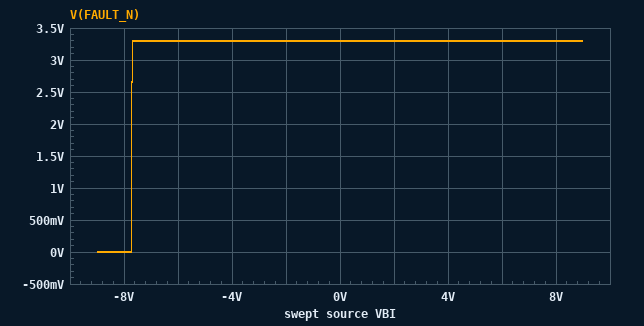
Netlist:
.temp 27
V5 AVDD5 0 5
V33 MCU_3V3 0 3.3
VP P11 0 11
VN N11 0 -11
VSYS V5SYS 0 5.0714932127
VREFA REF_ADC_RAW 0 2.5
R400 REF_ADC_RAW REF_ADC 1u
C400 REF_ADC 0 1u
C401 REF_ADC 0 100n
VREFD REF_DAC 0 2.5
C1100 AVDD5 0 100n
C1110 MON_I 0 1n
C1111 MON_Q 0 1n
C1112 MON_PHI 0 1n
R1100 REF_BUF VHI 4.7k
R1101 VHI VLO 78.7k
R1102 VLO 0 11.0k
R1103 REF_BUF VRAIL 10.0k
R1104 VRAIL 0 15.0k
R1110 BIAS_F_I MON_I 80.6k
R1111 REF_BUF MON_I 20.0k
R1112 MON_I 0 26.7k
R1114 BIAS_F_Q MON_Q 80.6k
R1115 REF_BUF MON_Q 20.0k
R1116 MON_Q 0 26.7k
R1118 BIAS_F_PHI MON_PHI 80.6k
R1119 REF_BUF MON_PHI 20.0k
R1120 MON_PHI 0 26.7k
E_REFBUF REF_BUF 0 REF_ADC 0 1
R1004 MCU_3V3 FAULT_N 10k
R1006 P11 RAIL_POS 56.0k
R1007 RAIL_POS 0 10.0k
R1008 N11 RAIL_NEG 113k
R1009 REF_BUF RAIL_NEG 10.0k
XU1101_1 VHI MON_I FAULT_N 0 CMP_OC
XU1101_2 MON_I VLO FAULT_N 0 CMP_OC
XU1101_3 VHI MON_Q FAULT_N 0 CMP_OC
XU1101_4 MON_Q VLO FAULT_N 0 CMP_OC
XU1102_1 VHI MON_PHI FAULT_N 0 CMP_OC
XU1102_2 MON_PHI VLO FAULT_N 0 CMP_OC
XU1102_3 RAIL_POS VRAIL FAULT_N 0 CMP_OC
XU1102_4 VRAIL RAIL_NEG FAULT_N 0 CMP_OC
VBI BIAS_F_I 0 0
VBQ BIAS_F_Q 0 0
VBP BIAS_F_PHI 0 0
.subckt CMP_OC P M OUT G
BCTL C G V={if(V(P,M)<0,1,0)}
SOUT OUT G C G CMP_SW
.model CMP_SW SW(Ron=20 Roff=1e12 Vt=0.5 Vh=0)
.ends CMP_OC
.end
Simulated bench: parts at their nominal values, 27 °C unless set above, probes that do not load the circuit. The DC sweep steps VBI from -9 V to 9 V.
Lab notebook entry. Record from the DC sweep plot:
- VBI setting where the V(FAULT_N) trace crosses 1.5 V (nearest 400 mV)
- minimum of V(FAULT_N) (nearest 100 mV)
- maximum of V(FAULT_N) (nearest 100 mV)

-7.6 V
0 V
3.3 V
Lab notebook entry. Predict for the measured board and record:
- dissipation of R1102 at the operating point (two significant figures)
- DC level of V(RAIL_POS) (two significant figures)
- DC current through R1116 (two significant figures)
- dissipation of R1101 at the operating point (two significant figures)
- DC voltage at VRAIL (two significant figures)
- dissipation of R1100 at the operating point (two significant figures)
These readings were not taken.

7.7 µW
1.7 V
47 µA
55 µW
1.5 V
3.3 µW
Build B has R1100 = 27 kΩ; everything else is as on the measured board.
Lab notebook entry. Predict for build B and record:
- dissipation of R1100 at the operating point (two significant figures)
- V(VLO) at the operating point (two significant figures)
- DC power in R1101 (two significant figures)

12 µW
240 mV
36 µW
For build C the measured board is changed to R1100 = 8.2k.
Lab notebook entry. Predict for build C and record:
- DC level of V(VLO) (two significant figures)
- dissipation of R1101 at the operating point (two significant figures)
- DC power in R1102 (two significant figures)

280 mV
51 µW
7.2 µW
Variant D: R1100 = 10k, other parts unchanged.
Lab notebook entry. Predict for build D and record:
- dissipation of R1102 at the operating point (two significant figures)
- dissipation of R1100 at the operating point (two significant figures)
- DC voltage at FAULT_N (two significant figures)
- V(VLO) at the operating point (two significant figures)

6.9 µW
6.3 µW
3.3 V
280 mV
